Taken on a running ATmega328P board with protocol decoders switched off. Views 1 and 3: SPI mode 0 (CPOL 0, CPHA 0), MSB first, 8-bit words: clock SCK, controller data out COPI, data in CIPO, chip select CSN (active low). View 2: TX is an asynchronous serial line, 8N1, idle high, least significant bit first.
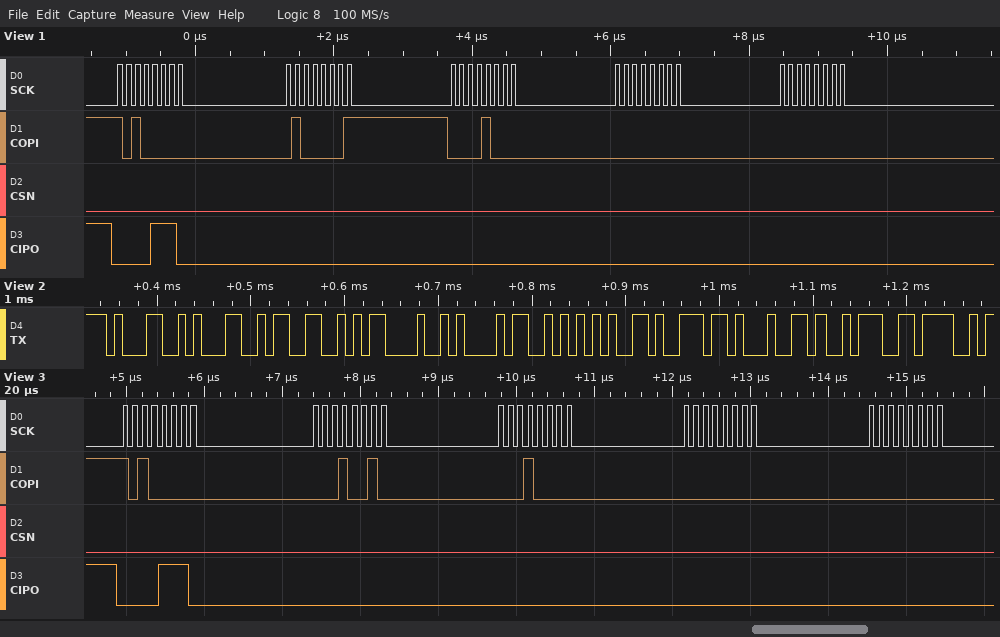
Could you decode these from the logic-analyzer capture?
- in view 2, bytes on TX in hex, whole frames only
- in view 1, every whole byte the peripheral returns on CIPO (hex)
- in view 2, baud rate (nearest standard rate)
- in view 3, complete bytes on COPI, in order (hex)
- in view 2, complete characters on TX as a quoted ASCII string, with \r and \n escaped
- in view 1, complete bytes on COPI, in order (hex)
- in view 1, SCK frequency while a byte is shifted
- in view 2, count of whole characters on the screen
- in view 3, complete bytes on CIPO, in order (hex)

0x31 0x31 0x33 0x0D 0x0A 0x53 0x65 0x6E 0x64 0x3A 0x4F
0E 00 00 00 00
115200 baud
A0 12 10 00 00
"113\r\nSend:O"
A0 41 08 00 00
8 MHz
11
0E 00 00 00 00
